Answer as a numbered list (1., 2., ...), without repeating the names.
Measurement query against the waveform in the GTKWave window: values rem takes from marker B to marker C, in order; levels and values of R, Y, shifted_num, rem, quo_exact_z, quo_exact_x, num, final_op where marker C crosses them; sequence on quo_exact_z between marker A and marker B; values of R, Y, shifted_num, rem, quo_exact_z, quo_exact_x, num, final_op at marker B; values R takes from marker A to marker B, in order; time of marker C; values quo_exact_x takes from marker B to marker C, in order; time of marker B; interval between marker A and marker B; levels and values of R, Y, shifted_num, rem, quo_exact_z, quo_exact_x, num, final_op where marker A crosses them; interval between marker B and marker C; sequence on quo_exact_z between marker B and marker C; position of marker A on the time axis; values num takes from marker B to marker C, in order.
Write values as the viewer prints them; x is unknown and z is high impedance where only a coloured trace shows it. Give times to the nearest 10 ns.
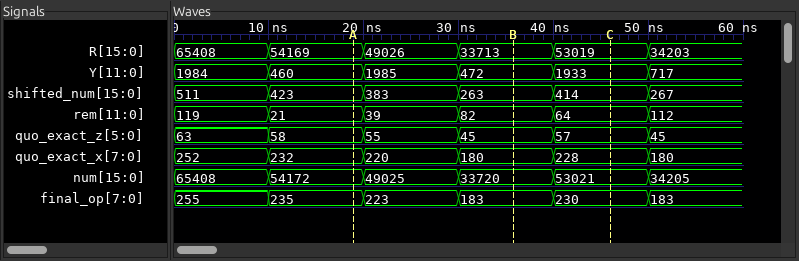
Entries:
1. 82, 64
2. R=53019, Y=1933, shifted_num=414, rem=64, quo_exact_z=57, quo_exact_x=228, num=53021, final_op=230
3. 58, 55, 45
4. R=33713, Y=472, shifted_num=263, rem=82, quo_exact_z=45, quo_exact_x=180, num=33720, final_op=183
5. 54169, 49026, 33713
6. 50 ns
7. 180, 228
8. 40 ns
9. 20 ns
10. R=54169, Y=460, shifted_num=423, rem=21, quo_exact_z=58, quo_exact_x=232, num=54172, final_op=235
11. 10 ns
12. 45, 57
13. 20 ns
14. 33720, 53021
